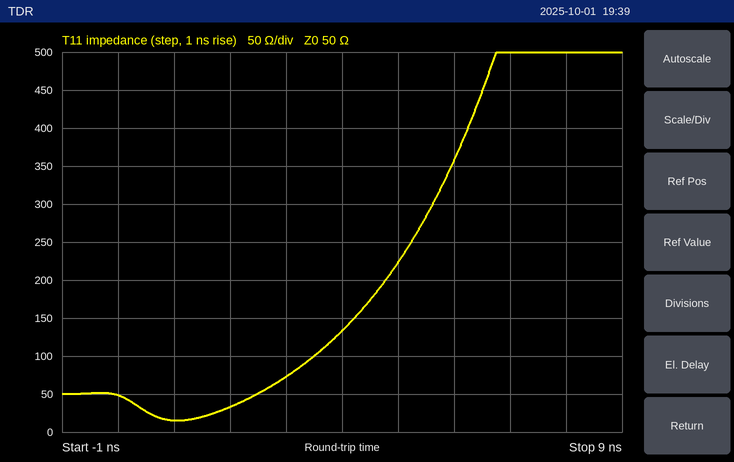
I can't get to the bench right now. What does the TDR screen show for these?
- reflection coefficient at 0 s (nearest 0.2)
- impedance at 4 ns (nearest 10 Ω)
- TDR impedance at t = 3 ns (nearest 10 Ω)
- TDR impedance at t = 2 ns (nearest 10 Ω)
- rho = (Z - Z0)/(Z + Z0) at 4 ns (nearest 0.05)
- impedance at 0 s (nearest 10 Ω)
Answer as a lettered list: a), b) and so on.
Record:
a) 0.0
b) 130 Ω
c) 70 Ω
d) 30 Ω
e) +0.45
f) 50 Ω
